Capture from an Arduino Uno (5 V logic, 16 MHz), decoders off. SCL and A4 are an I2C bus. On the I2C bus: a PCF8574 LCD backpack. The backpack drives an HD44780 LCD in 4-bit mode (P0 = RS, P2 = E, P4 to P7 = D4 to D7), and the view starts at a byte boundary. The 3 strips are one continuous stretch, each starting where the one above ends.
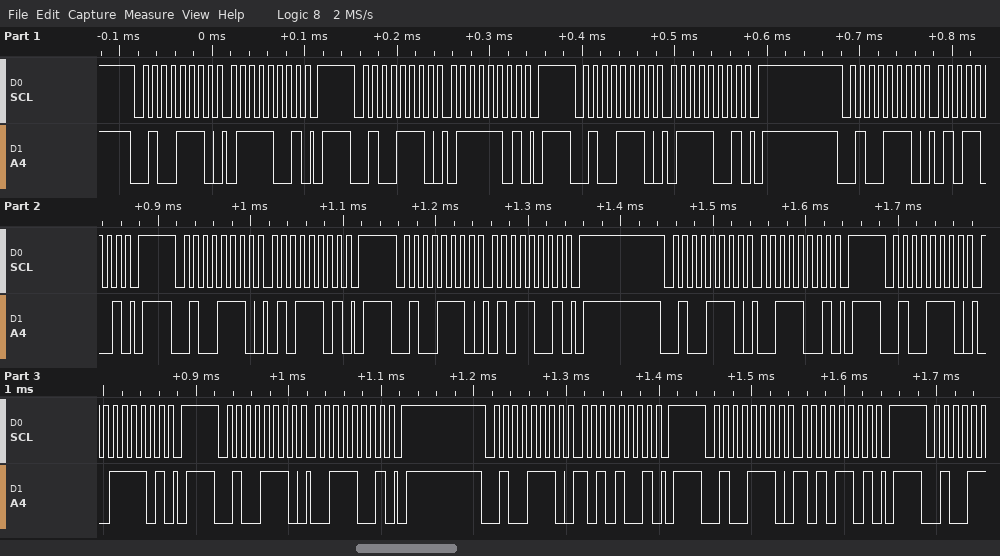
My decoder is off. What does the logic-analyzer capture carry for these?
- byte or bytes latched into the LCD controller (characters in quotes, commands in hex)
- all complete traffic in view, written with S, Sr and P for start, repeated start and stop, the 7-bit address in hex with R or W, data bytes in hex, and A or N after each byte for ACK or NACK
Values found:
'u'
S 27W A 79 A P S 27W A 7D A P S 27W A 79 A P S 27W A 59 A P S 27W A 5D A P S 27W A 59 A P S 27W A 39 A P S 27W A 3D A P S 27W A 39 A P S 27W A A9 A P S 27W A AD A P
